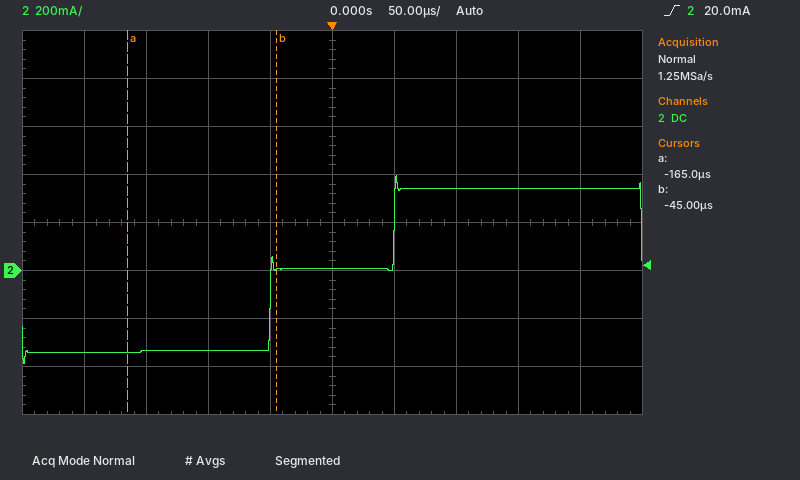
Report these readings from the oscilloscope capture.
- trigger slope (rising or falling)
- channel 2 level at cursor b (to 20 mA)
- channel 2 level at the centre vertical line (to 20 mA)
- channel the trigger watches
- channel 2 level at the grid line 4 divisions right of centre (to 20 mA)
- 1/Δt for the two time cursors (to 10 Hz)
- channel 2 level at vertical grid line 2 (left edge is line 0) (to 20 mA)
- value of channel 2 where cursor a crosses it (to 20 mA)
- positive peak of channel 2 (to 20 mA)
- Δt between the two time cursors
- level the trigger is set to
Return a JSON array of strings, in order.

["rising", "20 mA", "0 mA", "channel 2", "340 mA", "8.33 kHz", "-340 mA", "-340 mA", "400 mA", "120 µs", "20.0 mA"]
